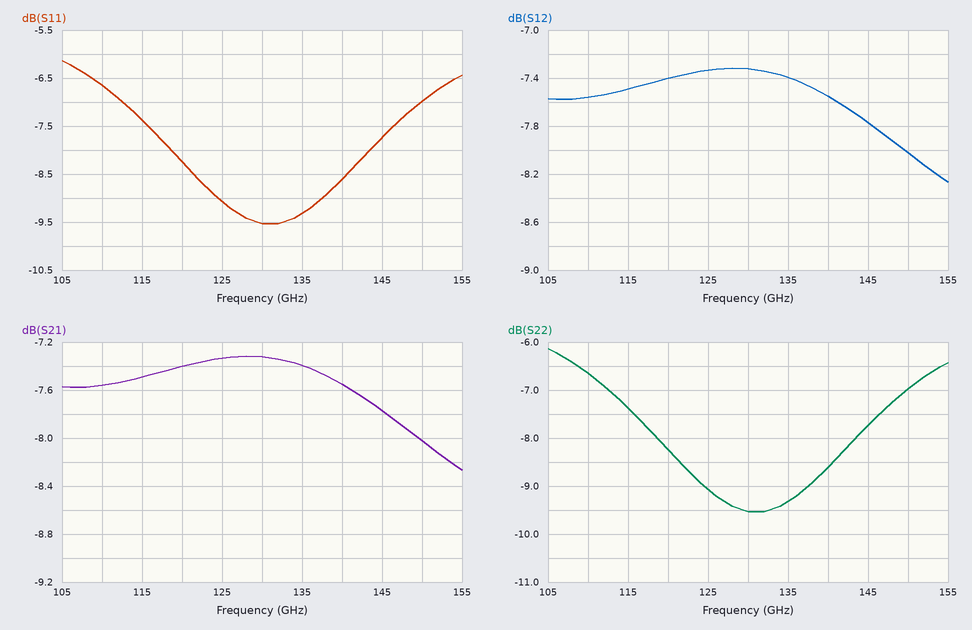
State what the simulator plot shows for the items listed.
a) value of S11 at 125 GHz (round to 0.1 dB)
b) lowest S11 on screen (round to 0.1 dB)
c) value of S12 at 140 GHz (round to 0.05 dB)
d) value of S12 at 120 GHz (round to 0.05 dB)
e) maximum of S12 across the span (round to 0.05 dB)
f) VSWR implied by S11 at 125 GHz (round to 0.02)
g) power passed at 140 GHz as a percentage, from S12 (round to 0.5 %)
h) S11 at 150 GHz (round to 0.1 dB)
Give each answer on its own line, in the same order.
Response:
-9.1 dB
-9.5 dB
-7.55 dB
-7.40 dB
-7.30 dB
2.08
17.5 %
-7.0 dB
